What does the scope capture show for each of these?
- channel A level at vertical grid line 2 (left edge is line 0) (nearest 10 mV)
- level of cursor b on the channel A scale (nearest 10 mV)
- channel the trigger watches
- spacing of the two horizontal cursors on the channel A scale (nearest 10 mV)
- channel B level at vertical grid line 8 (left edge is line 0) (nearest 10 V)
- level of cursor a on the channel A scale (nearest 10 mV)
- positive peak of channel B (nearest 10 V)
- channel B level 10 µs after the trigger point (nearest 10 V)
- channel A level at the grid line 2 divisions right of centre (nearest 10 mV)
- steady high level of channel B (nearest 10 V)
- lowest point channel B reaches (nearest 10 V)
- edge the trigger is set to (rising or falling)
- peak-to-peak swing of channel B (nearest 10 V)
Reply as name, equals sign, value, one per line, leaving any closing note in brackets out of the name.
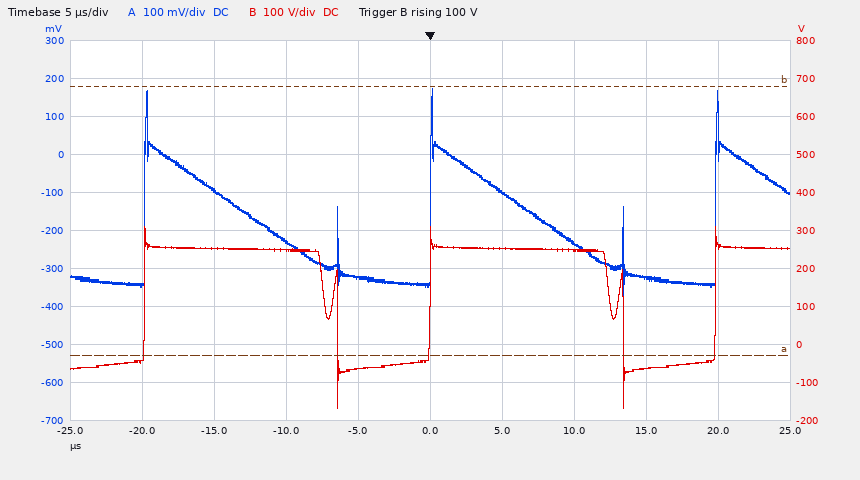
channel A level at vertical grid line 2 (left edge is line 0) = -100 mV
level of cursor b on the channel A scale = 180 mV
channel the trigger watches = channel B
spacing of the two horizontal cursors on the channel A scale = 710 mV
channel B level at vertical grid line 8 (left edge is line 0) = -60 V
level of cursor a on the channel A scale = -530 mV
positive peak of channel B = 310 V
channel B level 10 µs after the trigger point = 250 V
channel A level at the grid line 2 divisions right of centre = -230 mV
steady high level of channel B = 250 V
lowest point channel B reaches = -170 V
edge the trigger is set to = rising
peak-to-peak swing of channel B = 480 V
